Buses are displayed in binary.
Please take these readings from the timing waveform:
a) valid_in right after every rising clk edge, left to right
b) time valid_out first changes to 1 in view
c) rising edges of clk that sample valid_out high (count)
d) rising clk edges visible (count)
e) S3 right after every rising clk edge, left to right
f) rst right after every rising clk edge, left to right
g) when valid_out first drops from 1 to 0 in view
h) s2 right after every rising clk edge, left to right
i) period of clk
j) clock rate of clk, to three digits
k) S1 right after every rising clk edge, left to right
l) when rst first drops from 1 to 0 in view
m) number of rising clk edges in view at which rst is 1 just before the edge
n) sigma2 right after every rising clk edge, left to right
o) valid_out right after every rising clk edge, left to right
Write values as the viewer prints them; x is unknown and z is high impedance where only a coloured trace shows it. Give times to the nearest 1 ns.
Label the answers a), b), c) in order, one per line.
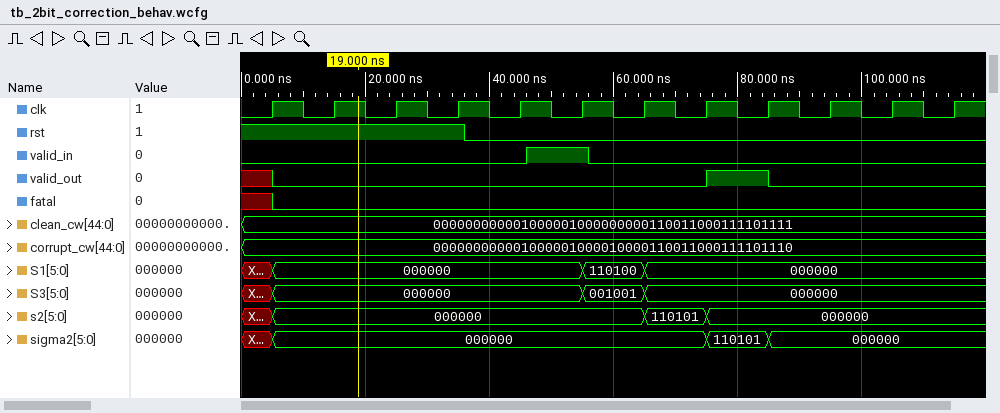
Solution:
a) 0 0 0 0 0 1 0 0 0 0 0 0
b) 75 ns
c) 1
d) 12
e) 000000, 000000, 000000, 000000, 000000, 001001, 000000, 000000, 000000, 000000, 000000, 000000
f) 1 1 1 1 0 0 0 0 0 0 0 0
g) 85 ns
h) 000000, 000000, 000000, 000000, 000000, 000000, 110101, 000000, 000000, 000000, 000000, 000000
i) 10 ns
j) 100 MHz
k) 000000, 000000, 000000, 000000, 000000, 110100, 000000, 000000, 000000, 000000, 000000, 000000
l) 36 ns
m) 4
n) 000000, 000000, 000000, 000000, 000000, 000000, 000000, 110101, 000000, 000000, 000000, 000000
o) 0 0 0 0 0 0 0 1 0 0 0 0
